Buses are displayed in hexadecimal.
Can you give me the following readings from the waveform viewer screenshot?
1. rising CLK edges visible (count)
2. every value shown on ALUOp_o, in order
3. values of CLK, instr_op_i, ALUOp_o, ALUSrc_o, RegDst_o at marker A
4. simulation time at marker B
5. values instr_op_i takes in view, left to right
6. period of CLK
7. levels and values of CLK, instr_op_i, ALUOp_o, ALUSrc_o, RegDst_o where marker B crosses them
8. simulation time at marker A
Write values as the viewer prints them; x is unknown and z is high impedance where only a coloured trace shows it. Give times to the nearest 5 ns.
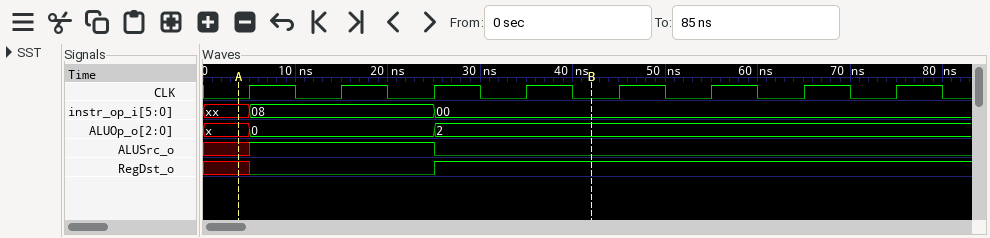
8
x, 0, 2
CLK=0, instr_op_i=xx, ALUOp_o=x, ALUSrc_o=x, RegDst_o=x
40 ns
xx, 08, 00
10 ns
CLK=0, instr_op_i=00, ALUOp_o=2, ALUSrc_o=0, RegDst_o=1
5 ns
